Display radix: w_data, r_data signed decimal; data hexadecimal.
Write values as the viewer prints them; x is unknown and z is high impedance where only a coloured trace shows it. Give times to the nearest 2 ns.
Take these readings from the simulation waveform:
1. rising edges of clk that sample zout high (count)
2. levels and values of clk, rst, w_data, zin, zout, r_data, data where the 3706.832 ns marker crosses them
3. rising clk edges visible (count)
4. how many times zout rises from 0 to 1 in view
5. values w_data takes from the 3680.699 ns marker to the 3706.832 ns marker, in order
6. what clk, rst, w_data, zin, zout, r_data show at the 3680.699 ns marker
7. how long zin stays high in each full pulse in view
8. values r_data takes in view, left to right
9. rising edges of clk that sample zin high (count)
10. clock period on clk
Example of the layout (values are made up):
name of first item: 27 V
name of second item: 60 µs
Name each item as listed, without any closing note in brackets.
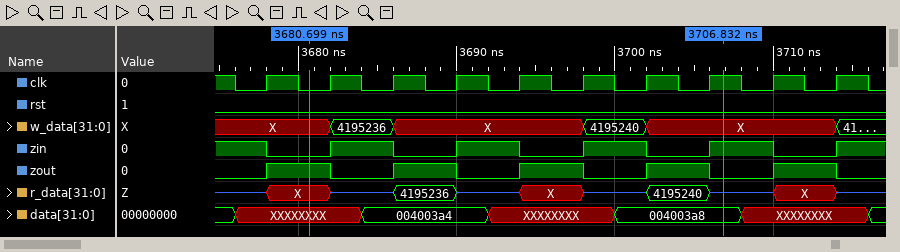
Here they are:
rising edges of clk that sample zout high: 5
levels and values of clk, rst, w_data, zin, zout, r_data, data where the 3706.832 ns marker crosses them: clk=1, rst=0, w_data=X, zin=1, zout=0, r_data=z, data=004003a8
rising clk edges visible: 10
how many times zout rises from 0 to 1 in view: 5
values w_data takes from the 3680.699 ns marker to the 3706.832 ns marker, in order: X, 4195236, X, 4195240, X
what clk, rst, w_data, zin, zout, r_data show at the 3680.699 ns marker: clk=0, rst=0, w_data=X, zin=0, zout=1, r_data=X
how long zin stays high in each full pulse in view: 4 ns, 4 ns, 4 ns, 4 ns
values r_data takes in view, left to right: z, X, z, 4195236, z, X, z, 4195240, z, X, z
rising edges of clk that sample zin high: 5
clock period on clk: 4 ns
